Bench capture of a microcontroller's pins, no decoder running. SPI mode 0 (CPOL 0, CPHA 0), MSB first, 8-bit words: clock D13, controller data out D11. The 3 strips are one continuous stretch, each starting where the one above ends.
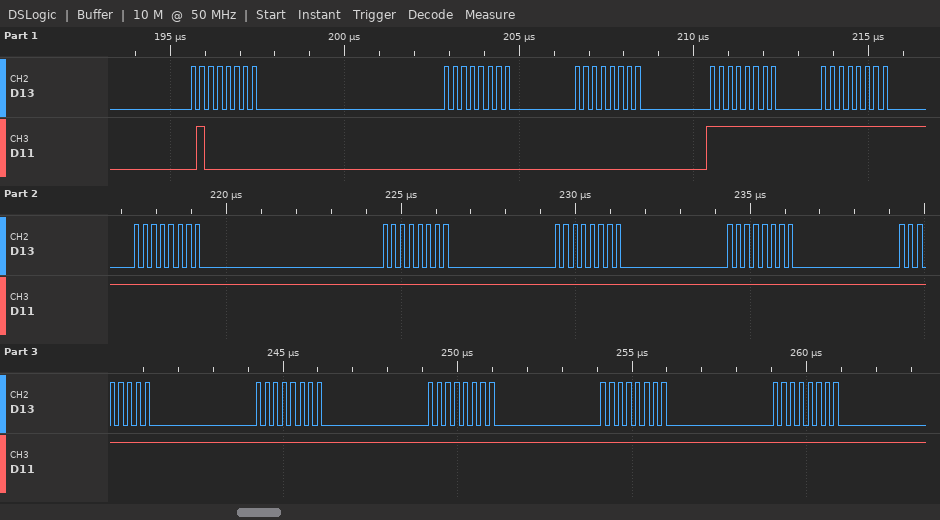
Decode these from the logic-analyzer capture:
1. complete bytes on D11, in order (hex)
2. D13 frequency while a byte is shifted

0x40 0x00 0x00 0xFF 0xFF 0xFF 0xFF 0xFF 0xFF 0xFF 0xFF 0xFF 0xFF 0xFF
4 MHz
